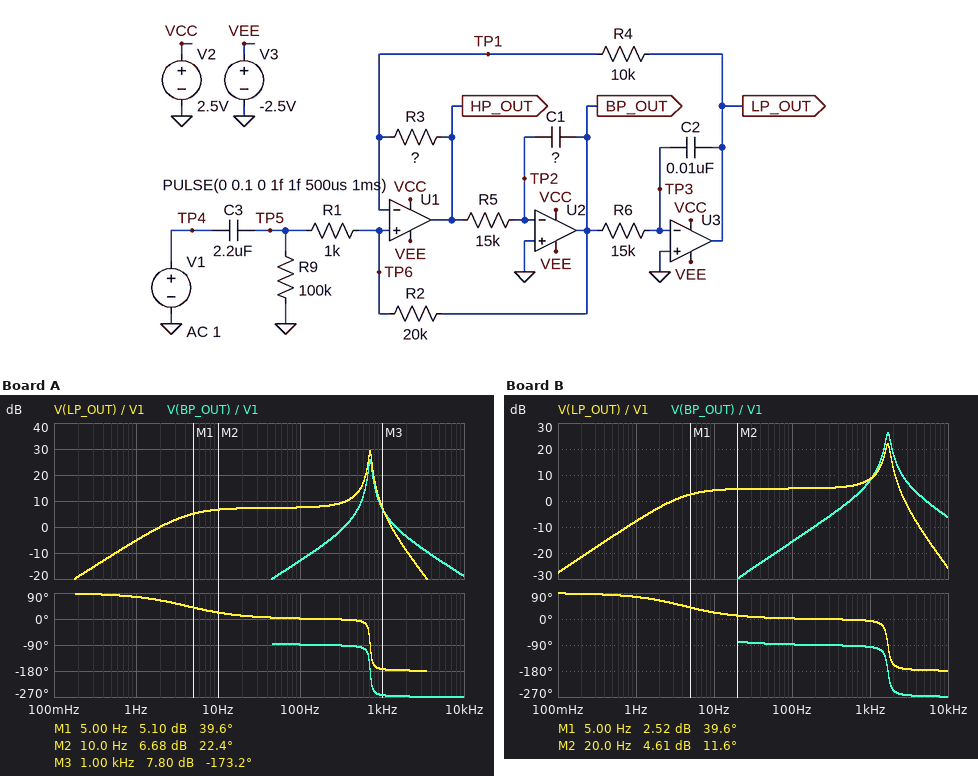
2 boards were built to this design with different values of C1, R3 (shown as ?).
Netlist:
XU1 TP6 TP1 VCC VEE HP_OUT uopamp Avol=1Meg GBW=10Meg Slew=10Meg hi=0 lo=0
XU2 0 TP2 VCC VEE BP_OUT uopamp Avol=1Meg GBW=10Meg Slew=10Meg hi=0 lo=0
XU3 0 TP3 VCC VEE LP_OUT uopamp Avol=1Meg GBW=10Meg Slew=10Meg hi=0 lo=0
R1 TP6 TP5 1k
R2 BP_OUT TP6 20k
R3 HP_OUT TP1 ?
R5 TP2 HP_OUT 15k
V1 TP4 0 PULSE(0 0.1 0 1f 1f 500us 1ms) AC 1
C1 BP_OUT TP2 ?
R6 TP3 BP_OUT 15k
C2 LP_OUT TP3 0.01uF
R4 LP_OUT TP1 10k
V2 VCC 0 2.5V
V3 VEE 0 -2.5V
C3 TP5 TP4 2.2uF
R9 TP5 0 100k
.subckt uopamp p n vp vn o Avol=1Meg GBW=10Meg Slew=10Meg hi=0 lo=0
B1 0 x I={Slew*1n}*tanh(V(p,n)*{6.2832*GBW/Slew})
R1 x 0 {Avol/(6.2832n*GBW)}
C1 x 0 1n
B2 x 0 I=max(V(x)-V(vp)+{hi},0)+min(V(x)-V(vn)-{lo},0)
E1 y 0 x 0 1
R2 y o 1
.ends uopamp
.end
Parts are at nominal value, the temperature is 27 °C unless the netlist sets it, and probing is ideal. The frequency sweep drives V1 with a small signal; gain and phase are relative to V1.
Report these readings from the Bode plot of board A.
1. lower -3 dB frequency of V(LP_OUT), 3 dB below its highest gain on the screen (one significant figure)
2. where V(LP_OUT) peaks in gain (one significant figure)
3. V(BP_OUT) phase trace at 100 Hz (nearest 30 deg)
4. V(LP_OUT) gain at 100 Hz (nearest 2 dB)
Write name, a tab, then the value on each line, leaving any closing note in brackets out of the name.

lower -3 dB frequency of V(LP_OUT), 3 dB below its highest gain on the screen	700 Hz
where V(LP_OUT) peaks in gain	700 Hz
V(BP_OUT) phase trace at 100 Hz	-90 deg
V(LP_OUT) gain at 100 Hz	8 dB
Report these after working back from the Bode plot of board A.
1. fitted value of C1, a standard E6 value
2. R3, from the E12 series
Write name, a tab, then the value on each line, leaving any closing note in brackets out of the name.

fitted value of C1, a standard E6 value	15 nF
R3, from the E12 series	6.8 kΩ
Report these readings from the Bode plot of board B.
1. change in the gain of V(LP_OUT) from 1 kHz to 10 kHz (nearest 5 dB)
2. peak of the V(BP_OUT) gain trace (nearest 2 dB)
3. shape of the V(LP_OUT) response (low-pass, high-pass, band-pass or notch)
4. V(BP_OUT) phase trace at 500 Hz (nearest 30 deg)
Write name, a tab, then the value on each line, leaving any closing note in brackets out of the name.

change in the gain of V(LP_OUT) from 1 kHz to 10 kHz	-35 dB
peak of the V(BP_OUT) gain trace	26 dB
shape of the V(LP_OUT) response	band-pass
V(BP_OUT) phase trace at 500 Hz	-90 deg
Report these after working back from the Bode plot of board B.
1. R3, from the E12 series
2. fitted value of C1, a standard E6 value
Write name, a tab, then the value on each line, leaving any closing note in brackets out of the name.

R3, from the E12 series	12 kΩ
fitted value of C1, a standard E6 value	4.7 nF
